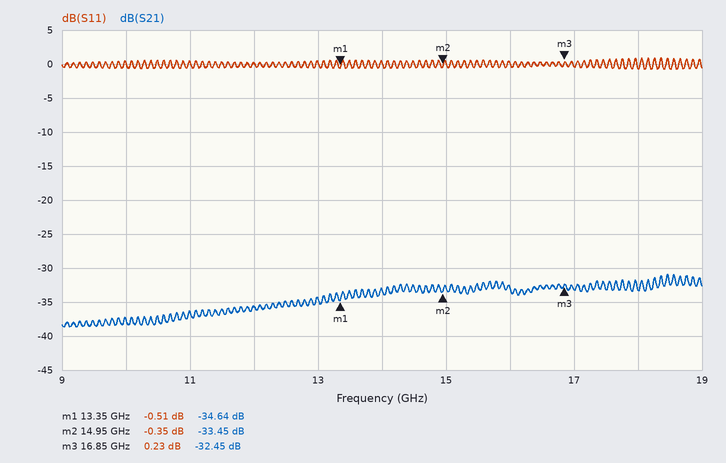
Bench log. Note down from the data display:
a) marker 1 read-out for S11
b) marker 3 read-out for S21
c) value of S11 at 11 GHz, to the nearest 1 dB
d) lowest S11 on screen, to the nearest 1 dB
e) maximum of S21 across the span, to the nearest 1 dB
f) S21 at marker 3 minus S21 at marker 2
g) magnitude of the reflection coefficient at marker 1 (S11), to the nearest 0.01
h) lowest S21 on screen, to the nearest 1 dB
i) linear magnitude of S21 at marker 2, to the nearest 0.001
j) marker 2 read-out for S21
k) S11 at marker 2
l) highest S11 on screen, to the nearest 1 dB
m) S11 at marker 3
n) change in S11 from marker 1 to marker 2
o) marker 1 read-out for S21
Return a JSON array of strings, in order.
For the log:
["-0.51 dB", "-32.45 dB", "0 dB", "-1 dB", "-31 dB", "1.00 dB", "0.94", "-39 dB", "0.021", "-33.45 dB", "-0.35 dB", "1 dB", "0.23 dB", "0.16 dB", "-34.64 dB"]
